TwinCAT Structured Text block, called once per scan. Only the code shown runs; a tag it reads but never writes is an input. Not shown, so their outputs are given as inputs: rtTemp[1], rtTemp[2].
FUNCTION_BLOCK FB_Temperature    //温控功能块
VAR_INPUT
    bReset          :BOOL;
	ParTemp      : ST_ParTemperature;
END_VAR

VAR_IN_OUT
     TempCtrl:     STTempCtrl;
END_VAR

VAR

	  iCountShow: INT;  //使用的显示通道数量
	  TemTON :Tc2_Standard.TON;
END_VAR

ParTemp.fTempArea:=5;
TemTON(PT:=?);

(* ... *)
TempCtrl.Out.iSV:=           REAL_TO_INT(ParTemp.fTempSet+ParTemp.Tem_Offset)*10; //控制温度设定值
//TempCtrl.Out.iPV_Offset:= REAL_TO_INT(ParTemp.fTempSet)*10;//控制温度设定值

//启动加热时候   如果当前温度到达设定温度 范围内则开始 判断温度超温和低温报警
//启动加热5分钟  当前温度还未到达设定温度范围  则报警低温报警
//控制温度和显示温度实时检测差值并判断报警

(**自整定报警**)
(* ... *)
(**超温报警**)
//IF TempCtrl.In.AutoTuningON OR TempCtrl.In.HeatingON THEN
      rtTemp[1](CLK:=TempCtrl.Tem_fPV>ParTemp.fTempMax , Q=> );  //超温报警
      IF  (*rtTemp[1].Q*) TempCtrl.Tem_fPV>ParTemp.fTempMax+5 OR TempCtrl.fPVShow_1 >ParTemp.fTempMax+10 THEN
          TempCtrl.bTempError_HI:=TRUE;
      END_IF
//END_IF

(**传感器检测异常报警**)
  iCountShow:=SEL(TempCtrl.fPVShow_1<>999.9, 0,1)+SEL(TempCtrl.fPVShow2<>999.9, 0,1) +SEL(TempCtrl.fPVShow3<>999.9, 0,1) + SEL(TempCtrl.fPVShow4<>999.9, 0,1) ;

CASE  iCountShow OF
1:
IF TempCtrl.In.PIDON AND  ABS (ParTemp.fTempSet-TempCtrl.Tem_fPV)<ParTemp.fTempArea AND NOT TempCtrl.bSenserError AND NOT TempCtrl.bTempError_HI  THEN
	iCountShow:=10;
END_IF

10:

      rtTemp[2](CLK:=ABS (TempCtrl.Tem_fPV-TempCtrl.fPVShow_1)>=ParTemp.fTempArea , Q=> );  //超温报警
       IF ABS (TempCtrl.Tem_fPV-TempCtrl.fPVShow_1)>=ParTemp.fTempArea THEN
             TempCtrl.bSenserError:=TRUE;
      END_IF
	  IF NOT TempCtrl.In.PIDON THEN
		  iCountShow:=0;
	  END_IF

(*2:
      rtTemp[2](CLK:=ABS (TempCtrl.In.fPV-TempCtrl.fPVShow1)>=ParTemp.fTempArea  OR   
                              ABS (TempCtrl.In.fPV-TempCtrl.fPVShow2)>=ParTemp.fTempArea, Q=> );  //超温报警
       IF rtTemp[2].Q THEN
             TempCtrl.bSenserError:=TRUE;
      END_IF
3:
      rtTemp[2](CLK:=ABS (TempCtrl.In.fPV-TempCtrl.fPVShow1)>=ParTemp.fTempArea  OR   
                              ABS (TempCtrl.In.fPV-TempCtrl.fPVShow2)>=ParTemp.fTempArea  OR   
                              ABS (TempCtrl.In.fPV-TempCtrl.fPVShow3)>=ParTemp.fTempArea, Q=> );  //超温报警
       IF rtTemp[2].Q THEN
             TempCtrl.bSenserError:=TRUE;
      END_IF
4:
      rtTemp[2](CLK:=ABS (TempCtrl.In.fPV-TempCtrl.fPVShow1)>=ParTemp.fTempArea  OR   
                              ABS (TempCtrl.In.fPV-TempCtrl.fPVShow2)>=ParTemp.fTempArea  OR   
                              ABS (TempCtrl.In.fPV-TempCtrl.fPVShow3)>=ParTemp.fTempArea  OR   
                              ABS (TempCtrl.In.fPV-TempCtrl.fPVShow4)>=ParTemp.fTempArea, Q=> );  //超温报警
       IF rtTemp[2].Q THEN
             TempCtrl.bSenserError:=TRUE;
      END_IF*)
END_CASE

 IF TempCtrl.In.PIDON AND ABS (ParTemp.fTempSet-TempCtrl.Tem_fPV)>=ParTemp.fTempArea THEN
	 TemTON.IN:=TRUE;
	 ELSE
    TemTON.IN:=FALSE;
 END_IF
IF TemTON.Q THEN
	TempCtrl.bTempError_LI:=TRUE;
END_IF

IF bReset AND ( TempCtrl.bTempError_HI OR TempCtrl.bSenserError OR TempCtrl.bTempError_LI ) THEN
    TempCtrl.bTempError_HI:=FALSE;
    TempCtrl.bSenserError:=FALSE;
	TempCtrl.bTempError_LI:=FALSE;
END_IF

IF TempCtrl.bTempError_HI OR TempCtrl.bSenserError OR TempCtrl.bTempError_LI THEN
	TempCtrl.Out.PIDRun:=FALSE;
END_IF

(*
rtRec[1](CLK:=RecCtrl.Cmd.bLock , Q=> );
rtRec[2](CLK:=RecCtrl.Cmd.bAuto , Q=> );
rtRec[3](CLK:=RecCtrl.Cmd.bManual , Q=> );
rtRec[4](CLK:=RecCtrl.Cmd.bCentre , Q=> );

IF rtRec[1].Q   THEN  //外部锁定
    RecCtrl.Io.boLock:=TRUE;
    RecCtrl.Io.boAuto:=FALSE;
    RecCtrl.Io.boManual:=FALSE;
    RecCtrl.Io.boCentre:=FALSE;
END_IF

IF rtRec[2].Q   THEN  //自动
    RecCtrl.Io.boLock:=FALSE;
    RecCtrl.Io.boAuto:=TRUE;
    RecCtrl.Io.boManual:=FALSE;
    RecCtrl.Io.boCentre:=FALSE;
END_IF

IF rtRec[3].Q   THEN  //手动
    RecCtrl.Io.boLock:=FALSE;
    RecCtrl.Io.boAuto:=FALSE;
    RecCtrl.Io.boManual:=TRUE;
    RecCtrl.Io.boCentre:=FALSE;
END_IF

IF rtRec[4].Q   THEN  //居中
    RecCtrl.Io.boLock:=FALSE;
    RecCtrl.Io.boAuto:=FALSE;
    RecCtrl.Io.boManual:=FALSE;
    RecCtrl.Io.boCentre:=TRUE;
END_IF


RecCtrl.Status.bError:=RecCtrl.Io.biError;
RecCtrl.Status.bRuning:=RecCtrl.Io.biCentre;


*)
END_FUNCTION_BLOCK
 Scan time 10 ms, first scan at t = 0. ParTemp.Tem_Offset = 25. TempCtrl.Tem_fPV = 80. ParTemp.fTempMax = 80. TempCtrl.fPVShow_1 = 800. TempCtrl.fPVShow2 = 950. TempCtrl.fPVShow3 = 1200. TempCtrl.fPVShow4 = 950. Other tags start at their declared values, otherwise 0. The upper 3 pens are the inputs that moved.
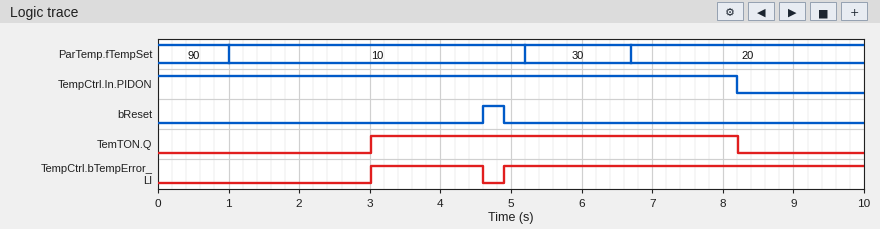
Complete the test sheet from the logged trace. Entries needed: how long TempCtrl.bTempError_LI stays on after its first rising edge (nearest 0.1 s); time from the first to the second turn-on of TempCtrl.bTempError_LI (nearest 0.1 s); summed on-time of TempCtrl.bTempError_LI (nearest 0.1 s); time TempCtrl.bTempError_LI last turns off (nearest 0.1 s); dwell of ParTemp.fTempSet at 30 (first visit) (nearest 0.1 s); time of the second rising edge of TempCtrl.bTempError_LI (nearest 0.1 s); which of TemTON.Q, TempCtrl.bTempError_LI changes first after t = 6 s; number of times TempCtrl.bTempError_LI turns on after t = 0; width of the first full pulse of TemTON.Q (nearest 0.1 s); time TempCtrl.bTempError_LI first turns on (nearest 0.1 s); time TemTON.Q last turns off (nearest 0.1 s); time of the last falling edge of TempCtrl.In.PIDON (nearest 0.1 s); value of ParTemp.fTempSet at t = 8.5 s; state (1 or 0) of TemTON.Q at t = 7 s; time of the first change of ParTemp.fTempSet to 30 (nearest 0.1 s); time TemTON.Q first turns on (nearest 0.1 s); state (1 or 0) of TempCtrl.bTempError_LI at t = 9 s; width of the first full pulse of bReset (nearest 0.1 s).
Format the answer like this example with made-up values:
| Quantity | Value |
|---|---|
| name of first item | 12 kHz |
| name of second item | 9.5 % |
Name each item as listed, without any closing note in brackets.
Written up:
| Quantity | Value |
|---|---|
| how long TempCtrl.bTempError_LI stays on after its first rising edge | 1.6 s |
| time from the first to the second turn-on of TempCtrl.bTempError_LI | 1.9 s |
| summed on-time of TempCtrl.bTempError_LI | 6.7 s |
| time TempCtrl.bTempError_LI last turns off | 4.6 s |
| dwell of ParTemp.fTempSet at 30 (first visit) | 1.5 s |
| time of the second rising edge of TempCtrl.bTempError_LI | 4.9 s |
| which of TemTON.Q, TempCtrl.bTempError_LI changes first after t = 6 s | TemTON.Q |
| number of times TempCtrl.bTempError_LI turns on after t = 0 | 2 |
| width of the first full pulse of TemTON.Q | 5.2 s |
| time TempCtrl.bTempError_LI first turns on | 3.0 s |
| time TemTON.Q last turns off | 8.2 s |
| time of the last falling edge of TempCtrl.In.PIDON | 8.2 s |
| value of ParTemp.fTempSet at t = 8.5 s | 20 |
| state (1 or 0) of TemTON.Q at t = 7 s | 1 |
| time of the first change of ParTemp.fTempSet to 30 | 5.2 s |
| time TemTON.Q first turns on | 3.0 s |
| state (1 or 0) of TempCtrl.bTempError_LI at t = 9 s | 1 |
| width of the first full pulse of bReset | 0.3 s |
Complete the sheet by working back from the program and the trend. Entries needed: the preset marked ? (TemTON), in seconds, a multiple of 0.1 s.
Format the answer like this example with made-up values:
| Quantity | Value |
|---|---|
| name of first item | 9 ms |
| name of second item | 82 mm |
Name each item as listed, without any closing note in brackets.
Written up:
| Quantity | Value |
|---|---|
| the preset marked ? (TemTON), in seconds, a multiple of 0.1 s | 3.0 s |
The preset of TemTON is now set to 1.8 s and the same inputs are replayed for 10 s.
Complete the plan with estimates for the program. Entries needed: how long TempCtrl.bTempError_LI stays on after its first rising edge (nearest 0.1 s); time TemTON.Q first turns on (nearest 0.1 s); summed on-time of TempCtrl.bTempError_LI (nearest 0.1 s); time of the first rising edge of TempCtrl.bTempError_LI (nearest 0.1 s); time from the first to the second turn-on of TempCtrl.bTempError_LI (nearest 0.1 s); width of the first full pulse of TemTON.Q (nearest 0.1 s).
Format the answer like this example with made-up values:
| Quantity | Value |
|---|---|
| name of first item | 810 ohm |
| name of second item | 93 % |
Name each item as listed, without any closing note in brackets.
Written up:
| Quantity | Value |
|---|---|
| how long TempCtrl.bTempError_LI stays on after its first rising edge | 2.8 s |
| time TemTON.Q first turns on | 1.8 s |
| summed on-time of TempCtrl.bTempError_LI | 7.9 s |
| time of the first rising edge of TempCtrl.bTempError_LI | 1.8 s |
| time from the first to the second turn-on of TempCtrl.bTempError_LI | 3.1 s |
| width of the first full pulse of TemTON.Q | 6.4 s |
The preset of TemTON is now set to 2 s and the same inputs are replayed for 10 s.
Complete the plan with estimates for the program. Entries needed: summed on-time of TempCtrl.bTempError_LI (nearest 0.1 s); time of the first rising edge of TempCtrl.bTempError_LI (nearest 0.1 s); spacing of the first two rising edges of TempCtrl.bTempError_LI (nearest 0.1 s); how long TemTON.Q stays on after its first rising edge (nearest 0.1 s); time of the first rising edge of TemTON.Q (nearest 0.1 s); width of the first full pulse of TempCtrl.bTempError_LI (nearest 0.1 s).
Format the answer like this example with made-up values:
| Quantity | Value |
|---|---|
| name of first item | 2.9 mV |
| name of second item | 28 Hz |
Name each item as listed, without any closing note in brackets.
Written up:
| Quantity | Value |
|---|---|
| summed on-time of TempCtrl.bTempError_LI | 7.7 s |
| time of the first rising edge of TempCtrl.bTempError_LI | 2.0 s |
| spacing of the first two rising edges of TempCtrl.bTempError_LI | 2.9 s |
| how long TemTON.Q stays on after its first rising edge | 6.2 s |
| time of the first rising edge of TemTON.Q | 2.0 s |
| width of the first full pulse of TempCtrl.bTempError_LI | 2.6 s |
